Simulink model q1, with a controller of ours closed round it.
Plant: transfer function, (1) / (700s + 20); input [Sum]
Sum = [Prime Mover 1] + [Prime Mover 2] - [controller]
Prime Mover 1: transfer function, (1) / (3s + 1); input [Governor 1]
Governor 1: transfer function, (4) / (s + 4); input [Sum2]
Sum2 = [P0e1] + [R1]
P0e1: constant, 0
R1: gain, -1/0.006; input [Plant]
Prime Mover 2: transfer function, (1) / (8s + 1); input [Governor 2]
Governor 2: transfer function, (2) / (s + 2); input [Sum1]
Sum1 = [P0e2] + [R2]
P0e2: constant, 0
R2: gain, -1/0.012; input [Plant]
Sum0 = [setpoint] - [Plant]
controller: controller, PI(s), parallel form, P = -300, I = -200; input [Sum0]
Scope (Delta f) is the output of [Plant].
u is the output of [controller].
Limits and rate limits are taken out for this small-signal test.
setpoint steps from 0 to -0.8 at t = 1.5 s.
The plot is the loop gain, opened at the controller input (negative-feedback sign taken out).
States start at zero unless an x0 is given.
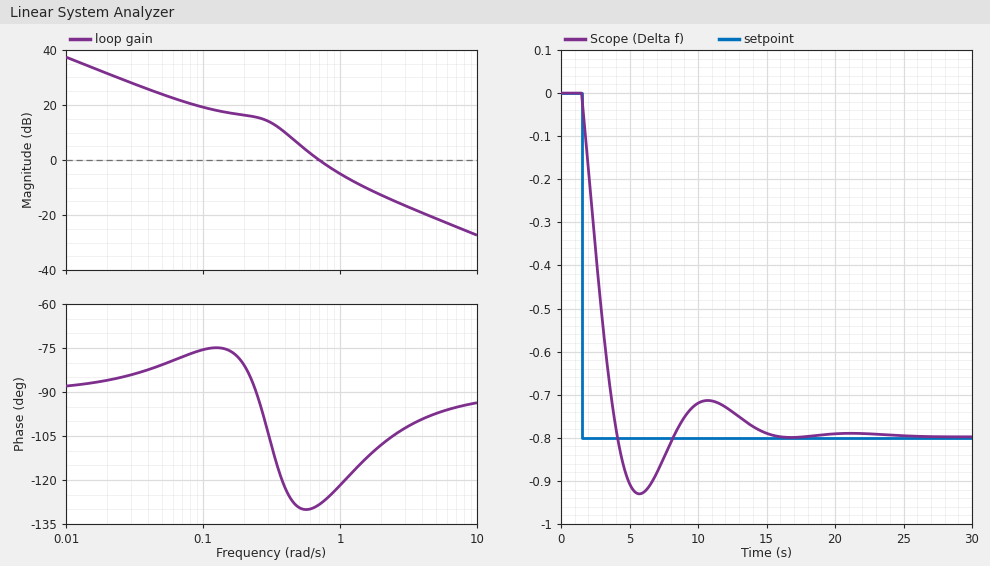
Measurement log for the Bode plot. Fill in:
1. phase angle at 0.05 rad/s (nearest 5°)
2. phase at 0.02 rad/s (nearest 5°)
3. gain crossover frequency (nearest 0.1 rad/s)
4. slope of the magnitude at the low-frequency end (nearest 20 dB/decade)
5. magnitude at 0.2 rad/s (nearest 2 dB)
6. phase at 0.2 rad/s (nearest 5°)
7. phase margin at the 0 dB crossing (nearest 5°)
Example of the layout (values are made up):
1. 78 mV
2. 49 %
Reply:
1. -80°
2. -85°
3. 0.7 rad/s
4. -20 dB/decade
5. 16 dB
6. -80°
7. 50°
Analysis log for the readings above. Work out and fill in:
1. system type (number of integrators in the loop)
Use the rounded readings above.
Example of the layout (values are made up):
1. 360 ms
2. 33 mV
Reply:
1. 1
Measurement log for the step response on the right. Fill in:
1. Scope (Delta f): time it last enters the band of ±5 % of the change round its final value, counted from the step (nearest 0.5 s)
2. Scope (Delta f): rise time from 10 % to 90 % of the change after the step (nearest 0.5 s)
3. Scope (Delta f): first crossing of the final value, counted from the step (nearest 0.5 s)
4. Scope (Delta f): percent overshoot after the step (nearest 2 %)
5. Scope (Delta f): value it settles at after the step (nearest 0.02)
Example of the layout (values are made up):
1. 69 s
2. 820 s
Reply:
1. 12.0 s
2. 2.0 s
3. 2.5 s
4. 16 %
5. -0.80
